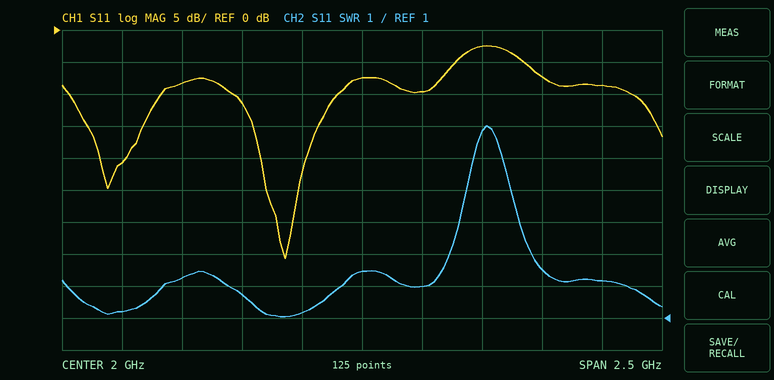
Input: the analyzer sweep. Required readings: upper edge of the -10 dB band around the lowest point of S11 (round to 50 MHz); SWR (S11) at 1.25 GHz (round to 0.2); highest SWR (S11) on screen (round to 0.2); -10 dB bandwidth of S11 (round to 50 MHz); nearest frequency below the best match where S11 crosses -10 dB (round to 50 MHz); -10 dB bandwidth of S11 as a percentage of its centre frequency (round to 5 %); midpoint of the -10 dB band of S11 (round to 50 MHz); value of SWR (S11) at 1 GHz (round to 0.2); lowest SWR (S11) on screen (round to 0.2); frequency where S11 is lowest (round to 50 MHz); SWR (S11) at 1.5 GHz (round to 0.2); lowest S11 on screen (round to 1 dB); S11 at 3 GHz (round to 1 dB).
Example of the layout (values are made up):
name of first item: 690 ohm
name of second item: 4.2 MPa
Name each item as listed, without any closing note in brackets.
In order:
upper edge of the -10 dB band around the lowest point of S11: 1.90 GHz
SWR (S11) at 1.25 GHz: 2.2
highest SWR (S11) on screen: 7.0
-10 dB bandwidth of S11: 450 MHz
nearest frequency below the best match where S11 crosses -10 dB: 1.45 GHz
-10 dB bandwidth of S11 as a percentage of its centre frequency: 25 %
midpoint of the -10 dB band of S11: 1.70 GHz
value of SWR (S11) at 1 GHz: 1.2
lowest SWR (S11) on screen: 1.0
frequency where S11 is lowest: 1.70 GHz
SWR (S11) at 1.5 GHz: 1.8
lowest S11 on screen: -36 dB
S11 at 3 GHz: -9 dB
